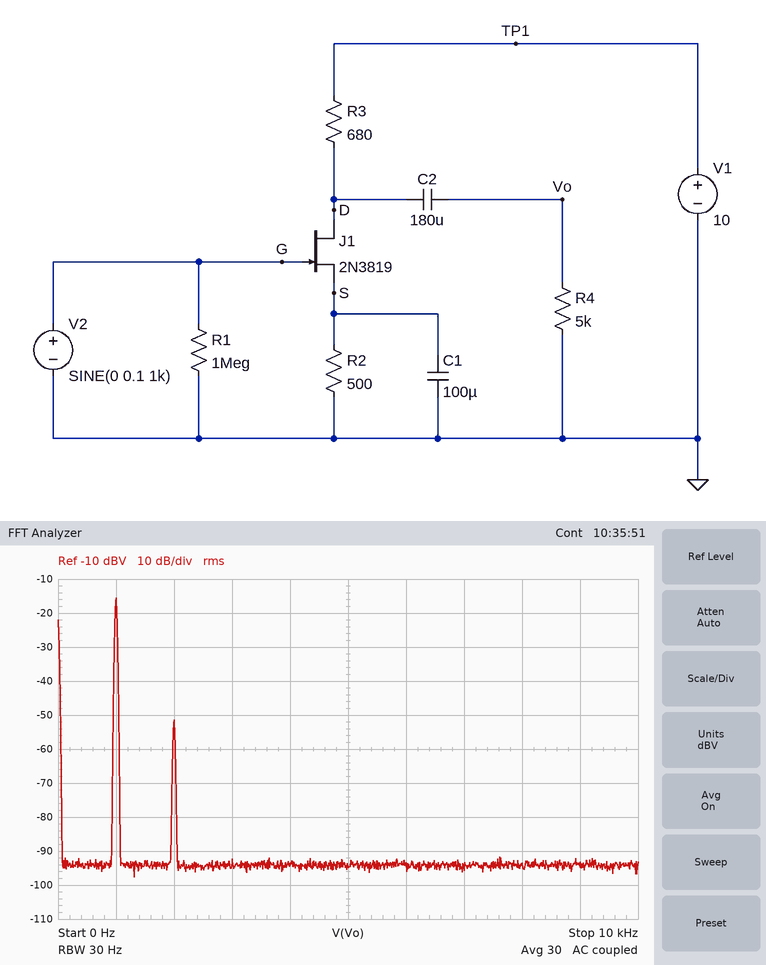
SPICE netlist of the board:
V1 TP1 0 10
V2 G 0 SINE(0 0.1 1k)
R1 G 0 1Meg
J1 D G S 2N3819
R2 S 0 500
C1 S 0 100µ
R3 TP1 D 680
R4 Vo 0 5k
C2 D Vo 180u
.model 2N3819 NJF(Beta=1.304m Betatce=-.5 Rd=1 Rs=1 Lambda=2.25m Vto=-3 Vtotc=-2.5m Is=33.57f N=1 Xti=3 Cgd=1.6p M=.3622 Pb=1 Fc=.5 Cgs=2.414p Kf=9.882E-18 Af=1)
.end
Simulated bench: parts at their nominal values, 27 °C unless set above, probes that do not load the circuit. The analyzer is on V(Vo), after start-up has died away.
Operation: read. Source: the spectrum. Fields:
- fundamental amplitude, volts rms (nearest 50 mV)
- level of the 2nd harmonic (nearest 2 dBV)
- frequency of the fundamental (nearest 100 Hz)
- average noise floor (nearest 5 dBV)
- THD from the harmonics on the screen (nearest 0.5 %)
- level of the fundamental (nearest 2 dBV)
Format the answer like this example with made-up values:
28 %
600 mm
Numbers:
150 mV
-52 dBV
1.0 kHz
-95 dBV
1.5 %
-16 dBV
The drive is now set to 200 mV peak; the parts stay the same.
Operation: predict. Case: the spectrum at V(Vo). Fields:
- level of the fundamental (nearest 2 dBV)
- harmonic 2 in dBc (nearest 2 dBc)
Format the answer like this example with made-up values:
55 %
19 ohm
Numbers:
-10 dBV
-30 dBc
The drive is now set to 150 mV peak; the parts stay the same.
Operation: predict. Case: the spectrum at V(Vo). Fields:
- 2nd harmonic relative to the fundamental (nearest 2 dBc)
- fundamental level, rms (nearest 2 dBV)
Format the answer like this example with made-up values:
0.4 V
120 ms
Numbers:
-32 dBc
-12 dBV
